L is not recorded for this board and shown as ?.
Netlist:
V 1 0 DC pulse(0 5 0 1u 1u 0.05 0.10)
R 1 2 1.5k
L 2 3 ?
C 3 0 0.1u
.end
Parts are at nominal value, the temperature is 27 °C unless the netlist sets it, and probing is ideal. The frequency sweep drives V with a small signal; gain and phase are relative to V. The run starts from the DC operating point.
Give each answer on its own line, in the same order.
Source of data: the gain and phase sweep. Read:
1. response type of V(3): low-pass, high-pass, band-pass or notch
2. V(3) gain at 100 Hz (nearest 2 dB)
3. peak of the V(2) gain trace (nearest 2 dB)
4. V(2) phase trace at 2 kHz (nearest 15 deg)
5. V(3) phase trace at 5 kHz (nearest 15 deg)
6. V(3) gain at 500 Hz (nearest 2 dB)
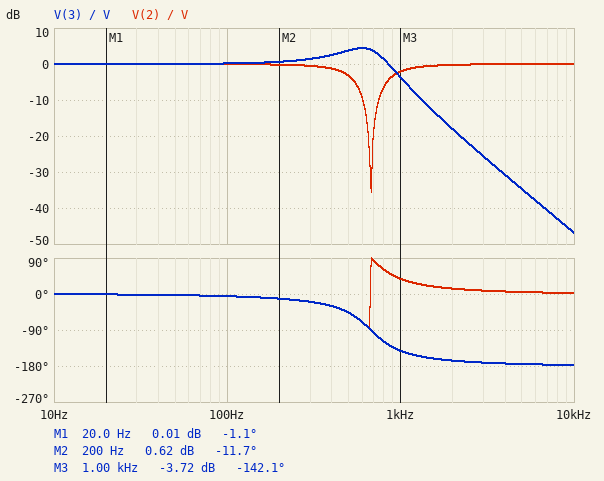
low-pass
0 dB
0 dB
15 deg
-180 deg
4 dB
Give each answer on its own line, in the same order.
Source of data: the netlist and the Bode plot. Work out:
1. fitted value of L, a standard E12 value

560 mH
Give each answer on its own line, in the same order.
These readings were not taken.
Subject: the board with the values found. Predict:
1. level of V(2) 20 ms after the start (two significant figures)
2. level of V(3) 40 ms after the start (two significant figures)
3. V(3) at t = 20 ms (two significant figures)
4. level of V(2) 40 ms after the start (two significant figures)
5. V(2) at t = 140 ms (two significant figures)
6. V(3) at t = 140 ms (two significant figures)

5.0 V
5.0 V
5.0 V
5.0 V
5.0 V
5.0 V
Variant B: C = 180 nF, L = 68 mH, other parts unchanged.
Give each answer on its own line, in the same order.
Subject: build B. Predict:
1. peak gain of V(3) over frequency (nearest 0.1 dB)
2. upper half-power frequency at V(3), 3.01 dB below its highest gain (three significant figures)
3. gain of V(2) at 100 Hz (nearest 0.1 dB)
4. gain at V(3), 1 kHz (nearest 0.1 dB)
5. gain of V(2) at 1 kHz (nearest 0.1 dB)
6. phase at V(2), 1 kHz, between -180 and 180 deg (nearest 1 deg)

0 dB
702 Hz
-0.1 dB
-5.0 dB
-10.7 dB
-73 deg
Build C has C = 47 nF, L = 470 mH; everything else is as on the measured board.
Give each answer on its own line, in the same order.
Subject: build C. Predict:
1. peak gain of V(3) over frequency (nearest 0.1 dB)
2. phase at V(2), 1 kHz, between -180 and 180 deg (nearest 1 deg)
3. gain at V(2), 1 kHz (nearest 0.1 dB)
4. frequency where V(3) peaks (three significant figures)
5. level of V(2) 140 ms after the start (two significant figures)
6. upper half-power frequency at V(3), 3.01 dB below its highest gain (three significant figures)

6.7 dB
-74 deg
-11.1 dB
1.01 kHz
5.0 V
1.24 kHz
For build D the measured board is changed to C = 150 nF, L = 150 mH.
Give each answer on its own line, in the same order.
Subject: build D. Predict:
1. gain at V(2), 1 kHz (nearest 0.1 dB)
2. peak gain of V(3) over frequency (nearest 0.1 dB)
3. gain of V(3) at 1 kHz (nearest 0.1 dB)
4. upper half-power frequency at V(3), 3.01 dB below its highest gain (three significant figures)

-22.1 dB
0 dB
-3.0 dB
997 Hz
